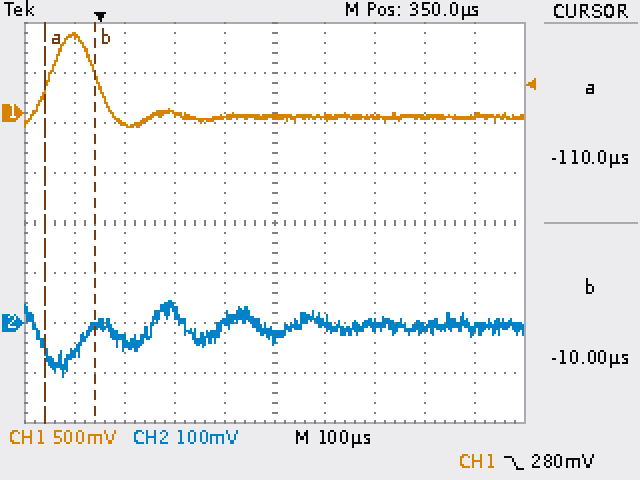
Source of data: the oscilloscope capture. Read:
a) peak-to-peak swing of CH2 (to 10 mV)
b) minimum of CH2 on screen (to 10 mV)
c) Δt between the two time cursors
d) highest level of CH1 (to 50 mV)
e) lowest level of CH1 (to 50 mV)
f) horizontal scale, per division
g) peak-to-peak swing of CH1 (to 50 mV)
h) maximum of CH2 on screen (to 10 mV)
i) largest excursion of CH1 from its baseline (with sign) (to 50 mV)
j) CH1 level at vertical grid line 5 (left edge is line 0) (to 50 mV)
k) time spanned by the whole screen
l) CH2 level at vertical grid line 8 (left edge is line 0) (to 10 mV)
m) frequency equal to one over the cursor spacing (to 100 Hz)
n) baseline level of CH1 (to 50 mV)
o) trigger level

150 mV
-110 mV
100 µs
800 mV
-150 mV
100 µs
950 mV
40 mV
+850 mV
-50 mV
1 ms
-10 mV
10.0 kHz
-50 mV
280 mV
